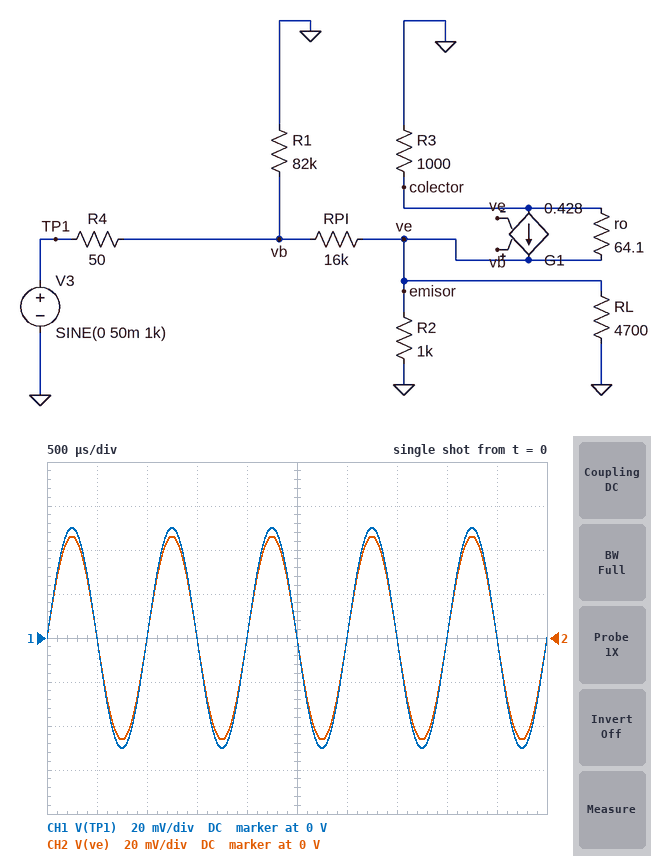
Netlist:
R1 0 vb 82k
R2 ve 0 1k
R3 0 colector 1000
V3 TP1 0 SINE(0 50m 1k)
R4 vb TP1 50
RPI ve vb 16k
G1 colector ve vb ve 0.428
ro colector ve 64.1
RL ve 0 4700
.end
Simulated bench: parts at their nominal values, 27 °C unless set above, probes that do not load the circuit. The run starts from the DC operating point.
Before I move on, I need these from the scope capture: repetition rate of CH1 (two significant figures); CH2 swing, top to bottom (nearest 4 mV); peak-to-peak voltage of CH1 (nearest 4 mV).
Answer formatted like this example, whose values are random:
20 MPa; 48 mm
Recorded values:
1.0 kHz; 92 mV; 100 mV
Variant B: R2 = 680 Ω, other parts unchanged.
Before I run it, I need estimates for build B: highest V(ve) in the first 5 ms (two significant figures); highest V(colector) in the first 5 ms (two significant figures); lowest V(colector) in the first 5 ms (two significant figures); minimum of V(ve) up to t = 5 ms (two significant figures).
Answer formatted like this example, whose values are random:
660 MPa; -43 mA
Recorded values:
45 mV; 76 mV; -76 mV; -45 mV
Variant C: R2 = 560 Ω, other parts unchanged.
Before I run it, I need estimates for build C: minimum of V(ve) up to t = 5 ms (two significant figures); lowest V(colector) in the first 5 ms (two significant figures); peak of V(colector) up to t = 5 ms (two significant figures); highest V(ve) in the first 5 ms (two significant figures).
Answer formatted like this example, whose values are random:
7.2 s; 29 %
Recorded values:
-45 mV; -89 mV; 89 mV; 45 mV
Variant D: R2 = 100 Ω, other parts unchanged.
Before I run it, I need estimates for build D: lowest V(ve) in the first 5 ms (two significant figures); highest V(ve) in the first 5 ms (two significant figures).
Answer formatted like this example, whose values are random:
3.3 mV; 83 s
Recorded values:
-35 mV; 35 mV
